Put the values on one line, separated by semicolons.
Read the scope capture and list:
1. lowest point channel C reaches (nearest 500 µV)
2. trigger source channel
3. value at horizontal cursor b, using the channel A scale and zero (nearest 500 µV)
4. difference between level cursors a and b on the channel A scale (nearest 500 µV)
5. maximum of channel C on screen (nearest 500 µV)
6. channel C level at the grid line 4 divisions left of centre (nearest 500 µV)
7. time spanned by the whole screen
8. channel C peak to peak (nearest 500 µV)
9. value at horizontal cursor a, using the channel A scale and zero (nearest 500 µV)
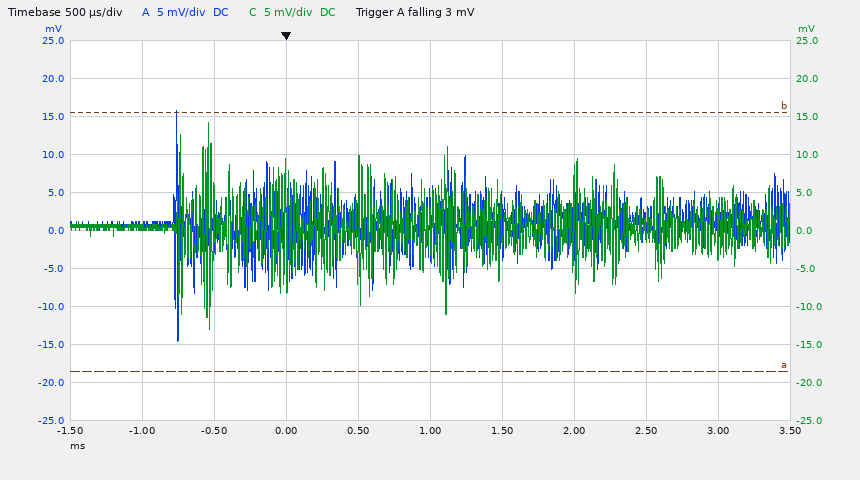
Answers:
-13.0 mV; channel A; 15.5 mV; 34.0 mV; 14.0 mV; 500 µV; 5 ms; 27.0 mV; -18.5 mV
